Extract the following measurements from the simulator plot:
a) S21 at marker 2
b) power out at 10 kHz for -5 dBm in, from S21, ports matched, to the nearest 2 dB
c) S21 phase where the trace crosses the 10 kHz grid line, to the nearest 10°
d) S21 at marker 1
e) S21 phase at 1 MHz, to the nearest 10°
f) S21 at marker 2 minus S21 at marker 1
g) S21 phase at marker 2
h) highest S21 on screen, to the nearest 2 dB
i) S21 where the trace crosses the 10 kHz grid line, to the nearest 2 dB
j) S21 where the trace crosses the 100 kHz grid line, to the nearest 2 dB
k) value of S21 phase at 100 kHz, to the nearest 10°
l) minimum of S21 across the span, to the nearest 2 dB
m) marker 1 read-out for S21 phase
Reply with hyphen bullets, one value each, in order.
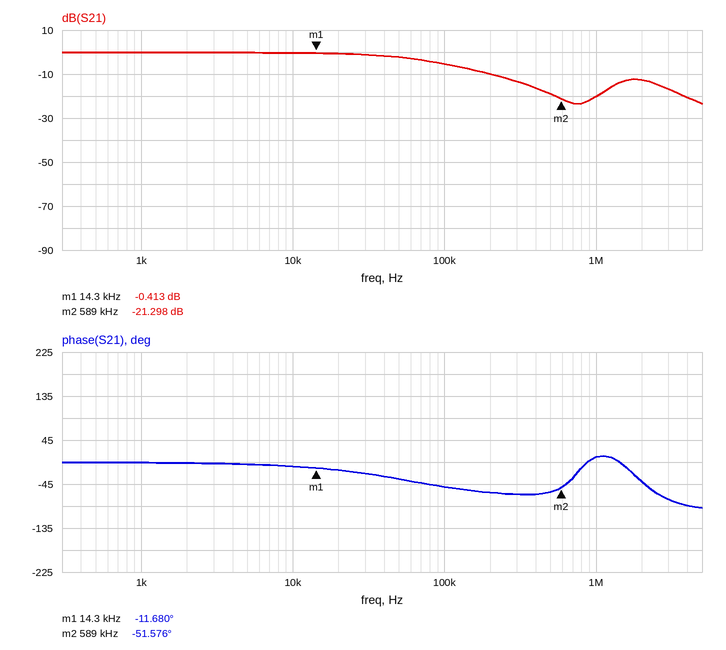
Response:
- -21.298 dB
- -6 dBm
- -10°
- -0.413 dB
- 10°
- -20.885 dB
- -51.576°
- 0 dB
- 0 dB
- -6 dB
- -50°
- -24 dB
- -11.680°
